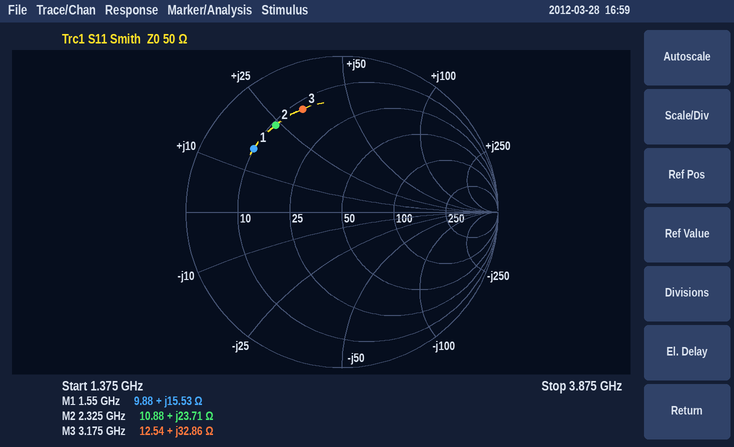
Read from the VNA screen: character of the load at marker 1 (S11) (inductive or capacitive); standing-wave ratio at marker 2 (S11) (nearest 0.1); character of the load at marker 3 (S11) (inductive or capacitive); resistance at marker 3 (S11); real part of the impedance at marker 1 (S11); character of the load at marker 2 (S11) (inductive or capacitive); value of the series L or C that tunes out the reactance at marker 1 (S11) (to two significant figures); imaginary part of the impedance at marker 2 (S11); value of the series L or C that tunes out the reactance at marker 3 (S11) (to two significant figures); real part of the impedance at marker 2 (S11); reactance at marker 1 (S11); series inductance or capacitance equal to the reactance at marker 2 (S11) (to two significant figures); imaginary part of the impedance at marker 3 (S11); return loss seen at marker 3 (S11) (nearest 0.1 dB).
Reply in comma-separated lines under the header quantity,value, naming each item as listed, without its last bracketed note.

quantity,value
character of the load at marker 1 (S11),inductive
standing-wave ratio at marker 2 (S11),5.7
character of the load at marker 3 (S11),inductive
resistance at marker 3,12.54 Ω
real part of the impedance at marker 1,9.88 Ω
character of the load at marker 2 (S11),inductive
value of the series L or C that tunes out the reactance at marker 1 (S11),6.6 pF
imaginary part of the impedance at marker 2,+23.71 Ω
value of the series L or C that tunes out the reactance at marker 3 (S11),1.5 pF
real part of the impedance at marker 2,10.88 Ω
reactance at marker 1,+15.53 Ω
series inductance or capacitance equal to the reactance at marker 2 (S11),1.6 nH
imaginary part of the impedance at marker 3,+32.86 Ω
return loss seen at marker 3 (S11),3.0 dB
